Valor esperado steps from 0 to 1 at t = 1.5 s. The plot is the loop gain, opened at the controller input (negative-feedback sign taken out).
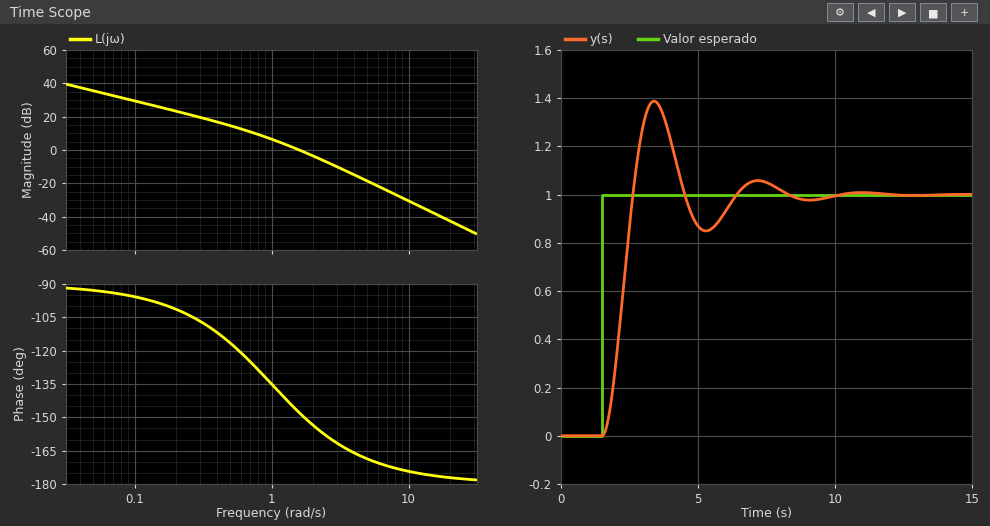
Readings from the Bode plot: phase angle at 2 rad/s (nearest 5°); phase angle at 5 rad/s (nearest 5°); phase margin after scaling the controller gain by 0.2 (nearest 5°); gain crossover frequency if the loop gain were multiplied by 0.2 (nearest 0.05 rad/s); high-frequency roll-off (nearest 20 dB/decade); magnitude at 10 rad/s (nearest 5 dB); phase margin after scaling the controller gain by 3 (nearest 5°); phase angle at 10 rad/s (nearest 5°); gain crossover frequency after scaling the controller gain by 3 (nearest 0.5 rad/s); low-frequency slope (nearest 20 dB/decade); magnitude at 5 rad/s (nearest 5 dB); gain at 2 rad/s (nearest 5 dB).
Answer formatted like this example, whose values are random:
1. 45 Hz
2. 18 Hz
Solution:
1. -155°
2. -170°
3. 60°
4. 0.55 rad/s
5. -40 dB/decade
6. -30 dB
7. 20°
8. -175°
9. 3.0 rad/s
10. -20 dB/decade
11. -20 dB
12. -5 dB
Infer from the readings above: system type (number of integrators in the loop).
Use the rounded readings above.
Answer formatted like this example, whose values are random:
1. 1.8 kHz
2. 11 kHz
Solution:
1. 1
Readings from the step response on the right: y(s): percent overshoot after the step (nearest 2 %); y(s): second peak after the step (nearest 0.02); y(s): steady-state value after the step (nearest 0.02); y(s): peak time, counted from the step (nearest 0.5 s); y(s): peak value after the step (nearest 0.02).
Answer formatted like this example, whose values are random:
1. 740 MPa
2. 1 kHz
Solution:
1. 38 %
2. 1.06
3. 1.00
4. 2.0 s
5. 1.38
